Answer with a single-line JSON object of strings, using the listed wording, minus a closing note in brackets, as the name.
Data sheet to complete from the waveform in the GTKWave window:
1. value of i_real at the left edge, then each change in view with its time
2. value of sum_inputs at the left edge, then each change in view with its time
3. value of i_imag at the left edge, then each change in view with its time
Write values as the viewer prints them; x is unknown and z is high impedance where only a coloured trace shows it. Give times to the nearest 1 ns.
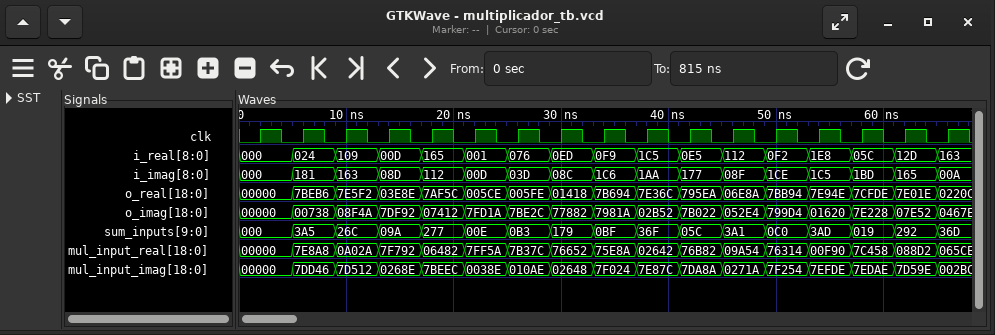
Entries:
{"value of i_real at the left edge, then each change in view with its time": "000, 024 at 5 ns, 109 at 9 ns, 00D at 13 ns, 165 at 17 ns, 001 at 21 ns, 076 at 25 ns, 0ED at 29 ns, 0F9 at 33 ns, 1C5 at 37 ns, 0E5 at 41 ns, 112 at 45 ns, 0F2 at 49 ns, 1E8 at 53 ns, 05C at 57 ns, 12D at 61 ns, 163 at 65 ns", "value of sum_inputs at the left edge, then each change in view with its time": "000, 3A5 at 5 ns, 26C at 9 ns, 09A at 13 ns, 277 at 17 ns, 00E at 21 ns, 0B3 at 25 ns, 179 at 29 ns, 0BF at 33 ns, 36F at 37 ns, 05C at 41 ns, 3A1 at 45 ns, 0C0 at 49 ns, 3AD at 53 ns, 019 at 57 ns, 292 at 61 ns, 36D at 65 ns", "value of i_imag at the left edge, then each change in view with its time": "000, 181 at 5 ns, 163 at 9 ns, 08D at 13 ns, 112 at 17 ns, 00D at 21 ns, 03D at 25 ns, 08C at 29 ns, 1C6 at 33 ns, 1AA at 37 ns, 177 at 41 ns, 08F at 45 ns, 1CE at 49 ns, 1C5 at 53 ns, 1BD at 57 ns, 165 at 61 ns, 00A at 65 ns"}
